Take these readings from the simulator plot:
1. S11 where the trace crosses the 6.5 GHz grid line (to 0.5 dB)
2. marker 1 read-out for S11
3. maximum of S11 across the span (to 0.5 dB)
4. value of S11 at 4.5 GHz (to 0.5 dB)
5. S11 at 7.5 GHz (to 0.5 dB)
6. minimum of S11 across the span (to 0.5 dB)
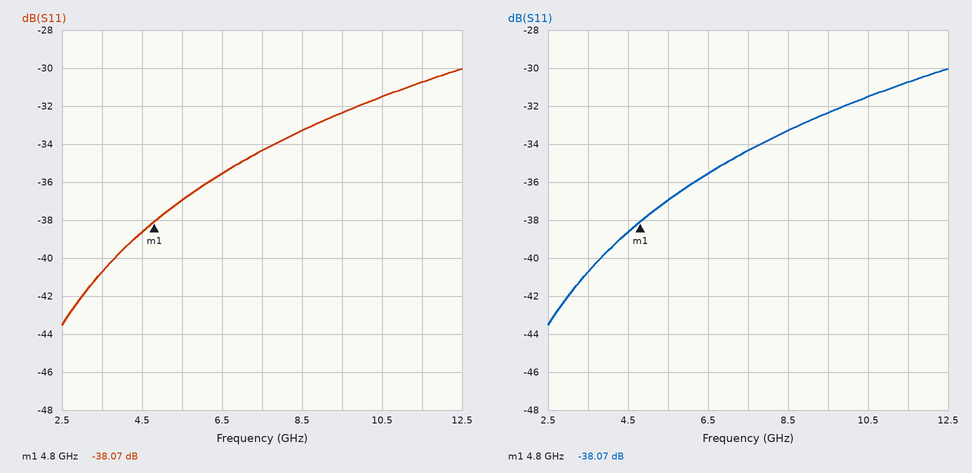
-35.5 dB
-38.07 dB
-30.0 dB
-38.5 dB
-34.5 dB
-43.5 dB
